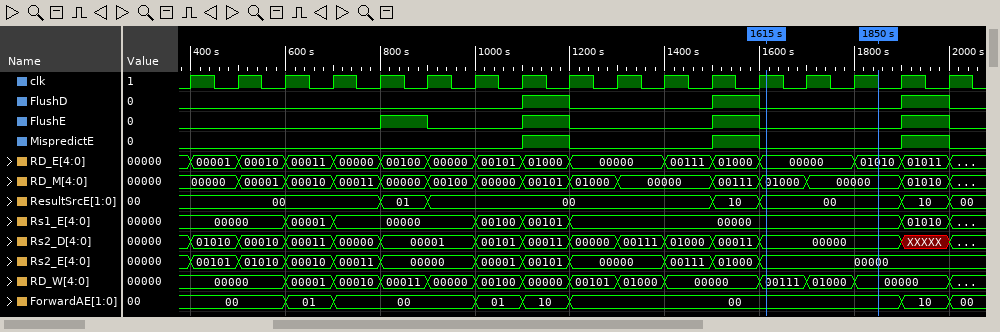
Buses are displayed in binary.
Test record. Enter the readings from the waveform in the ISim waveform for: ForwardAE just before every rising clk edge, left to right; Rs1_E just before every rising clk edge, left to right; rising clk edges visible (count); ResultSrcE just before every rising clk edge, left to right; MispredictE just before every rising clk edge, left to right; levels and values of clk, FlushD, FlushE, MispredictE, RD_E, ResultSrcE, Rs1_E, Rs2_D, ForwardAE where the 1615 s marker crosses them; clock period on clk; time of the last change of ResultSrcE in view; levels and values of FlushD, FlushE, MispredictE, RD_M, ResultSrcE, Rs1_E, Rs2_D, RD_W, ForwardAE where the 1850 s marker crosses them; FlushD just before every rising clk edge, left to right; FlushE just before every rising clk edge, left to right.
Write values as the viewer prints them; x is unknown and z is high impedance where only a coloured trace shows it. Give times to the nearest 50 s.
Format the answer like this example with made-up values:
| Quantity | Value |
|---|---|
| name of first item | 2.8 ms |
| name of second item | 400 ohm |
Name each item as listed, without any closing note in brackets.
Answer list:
| Quantity | Value |
|---|---|
| ForwardAE just before every rising clk edge, left to right | 00, 00, 00, 01, 00, 00, 00, 01, 10, 00, 00, 00, 00, 00, 00, 00, 10 |
| Rs1_E just before every rising clk edge, left to right | 00000, 00000, 00000, 00001, 00000, 00000, 00000, 00100, 00101, 00000, 00000, 00000, 00000, 00000, 00000, 00000, 01010 |
| rising clk edges visible | 17 |
| ResultSrcE just before every rising clk edge, left to right | 00, 00, 00, 00, 00, 01, 00, 00, 00, 00, 00, 00, 10, 00, 00, 00, 10 |
| MispredictE just before every rising clk edge, left to right | 0 0 0 0 0 0 0 0 1 0 0 0 1 0 0 0 1 |
| levels and values of clk, FlushD, FlushE, MispredictE, RD_E, ResultSrcE, Rs1_E, Rs2_D, ForwardAE where the 1615 s marker crosses them | clk=1, FlushD=0, FlushE=0, MispredictE=0, RD_E=00000, ResultSrcE=00, Rs1_E=00000, Rs2_D=00000, ForwardAE=00 |
| clock period on clk | 100 s |
| time of the last change of ResultSrcE in view | 2000 s |
| levels and values of FlushD, FlushE, MispredictE, RD_M, ResultSrcE, Rs1_E, Rs2_D, RD_W, ForwardAE where the 1850 s marker crosses them | FlushD=0, FlushE=0, MispredictE=0, RD_M=00000, ResultSrcE=00, Rs1_E=00000, Rs2_D=00000, RD_W=00000, ForwardAE=00 |
| FlushD just before every rising clk edge, left to right | 0 0 0 0 0 0 0 0 1 0 0 0 1 0 0 0 1 |
| FlushE just before every rising clk edge, left to right | 0 0 0 0 0 1 0 0 1 0 0 0 1 0 0 0 1 |
